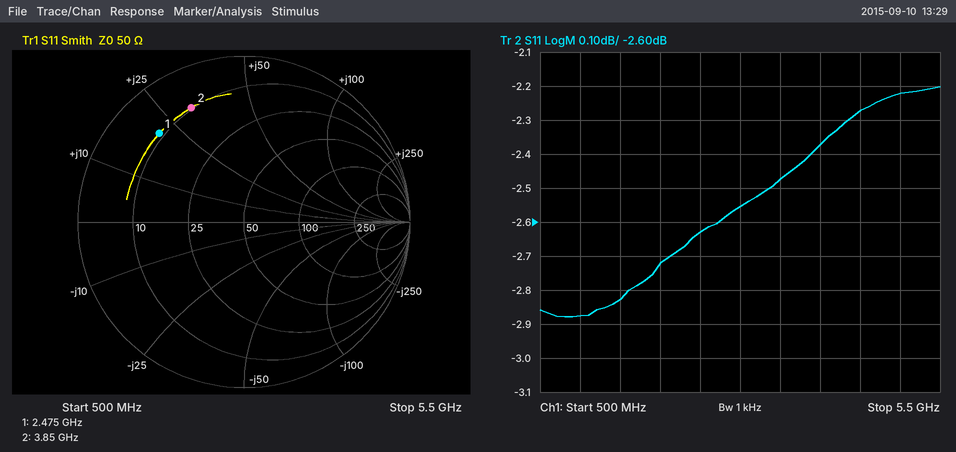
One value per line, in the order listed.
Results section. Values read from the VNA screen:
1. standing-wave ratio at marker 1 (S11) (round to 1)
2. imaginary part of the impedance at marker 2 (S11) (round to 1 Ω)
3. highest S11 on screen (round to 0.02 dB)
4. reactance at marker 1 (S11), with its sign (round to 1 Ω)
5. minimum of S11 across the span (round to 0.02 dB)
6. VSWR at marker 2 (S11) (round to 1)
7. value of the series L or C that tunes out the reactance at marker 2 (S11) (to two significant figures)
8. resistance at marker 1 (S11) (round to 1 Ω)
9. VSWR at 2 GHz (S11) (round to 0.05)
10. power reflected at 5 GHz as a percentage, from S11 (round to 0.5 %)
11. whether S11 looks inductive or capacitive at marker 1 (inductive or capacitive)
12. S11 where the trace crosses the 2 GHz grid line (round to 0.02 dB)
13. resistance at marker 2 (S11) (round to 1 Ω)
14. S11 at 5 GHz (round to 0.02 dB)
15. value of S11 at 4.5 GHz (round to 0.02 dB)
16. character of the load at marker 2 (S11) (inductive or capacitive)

7
+31 Ω
-2.20 dB
+21 Ω
-2.88 dB
7
1.3 pF
9 Ω
6.45
60.0 %
inductive
-2.72 dB
10 Ω
-2.22 dB
-2.28 dB
inductive
